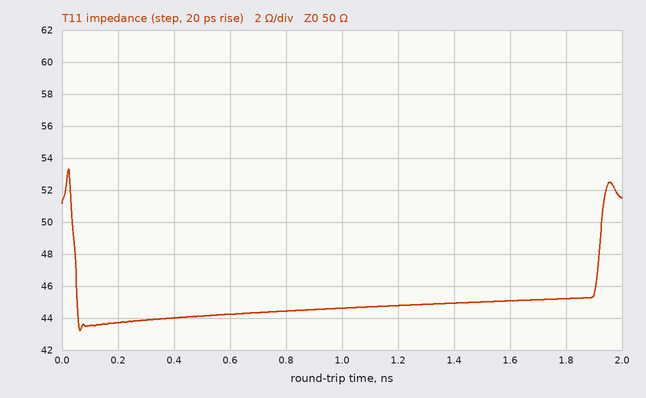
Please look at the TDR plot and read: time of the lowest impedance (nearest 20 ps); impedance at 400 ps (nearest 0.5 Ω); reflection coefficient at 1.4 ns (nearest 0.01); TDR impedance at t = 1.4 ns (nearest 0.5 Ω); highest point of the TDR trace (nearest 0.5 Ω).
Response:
60 ps
44.0 Ω
-0.05
45.0 Ω
53.5 Ω
